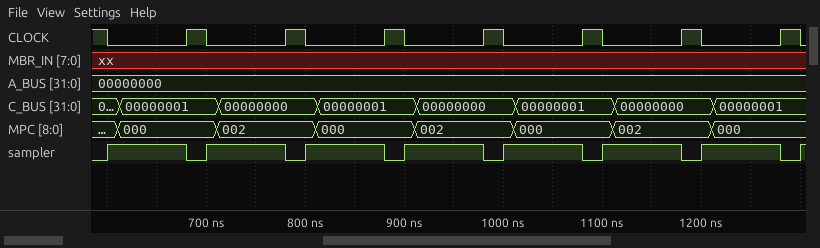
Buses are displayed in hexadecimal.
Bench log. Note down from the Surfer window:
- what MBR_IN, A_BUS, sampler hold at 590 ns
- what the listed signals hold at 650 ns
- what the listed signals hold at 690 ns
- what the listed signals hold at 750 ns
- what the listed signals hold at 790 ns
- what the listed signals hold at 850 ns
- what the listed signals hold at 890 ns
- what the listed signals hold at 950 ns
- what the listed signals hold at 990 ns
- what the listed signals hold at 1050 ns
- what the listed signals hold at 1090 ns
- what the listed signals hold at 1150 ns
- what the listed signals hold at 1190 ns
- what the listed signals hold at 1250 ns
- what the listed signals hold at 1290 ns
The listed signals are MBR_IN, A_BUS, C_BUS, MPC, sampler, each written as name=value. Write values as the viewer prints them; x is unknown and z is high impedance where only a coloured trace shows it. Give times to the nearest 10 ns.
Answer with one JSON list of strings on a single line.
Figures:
["MBR_IN=xx, A_BUS=00000000, sampler=0", "MBR_IN=xx, A_BUS=00000000, C_BUS=00000001, MPC=000, sampler=1", "MBR_IN=xx, A_BUS=00000000, C_BUS=00000001, MPC=000, sampler=0", "MBR_IN=xx, A_BUS=00000000, C_BUS=00000000, MPC=002, sampler=1", "MBR_IN=xx, A_BUS=00000000, C_BUS=00000000, MPC=002, sampler=0", "MBR_IN=xx, A_BUS=00000000, C_BUS=00000001, MPC=000, sampler=1", "MBR_IN=xx, A_BUS=00000000, C_BUS=00000001, MPC=000, sampler=0", "MBR_IN=xx, A_BUS=00000000, C_BUS=00000000, MPC=002, sampler=1", "MBR_IN=xx, A_BUS=00000000, C_BUS=00000000, MPC=002, sampler=0", "MBR_IN=xx, A_BUS=00000000, C_BUS=00000001, MPC=000, sampler=1", "MBR_IN=xx, A_BUS=00000000, C_BUS=00000001, MPC=000, sampler=0", "MBR_IN=xx, A_BUS=00000000, C_BUS=00000000, MPC=002, sampler=1", "MBR_IN=xx, A_BUS=00000000, C_BUS=00000000, MPC=002, sampler=0", "MBR_IN=xx, A_BUS=00000000, C_BUS=00000001, MPC=000, sampler=1", "MBR_IN=xx, A_BUS=00000000, C_BUS=00000001, MPC=000, sampler=0"]
